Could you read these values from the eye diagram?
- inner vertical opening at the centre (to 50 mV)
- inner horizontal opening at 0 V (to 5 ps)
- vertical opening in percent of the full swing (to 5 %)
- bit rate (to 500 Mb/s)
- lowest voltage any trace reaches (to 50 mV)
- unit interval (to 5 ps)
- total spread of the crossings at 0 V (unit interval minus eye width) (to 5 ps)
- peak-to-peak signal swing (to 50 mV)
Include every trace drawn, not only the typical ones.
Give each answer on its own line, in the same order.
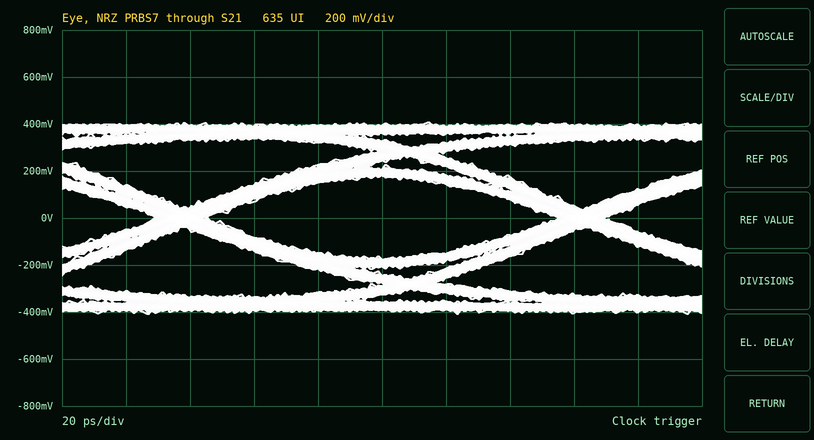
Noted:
350 mV
110 ps
45 %
8.0 Gb/s
-400 mV
125 ps
15 ps
800 mV
